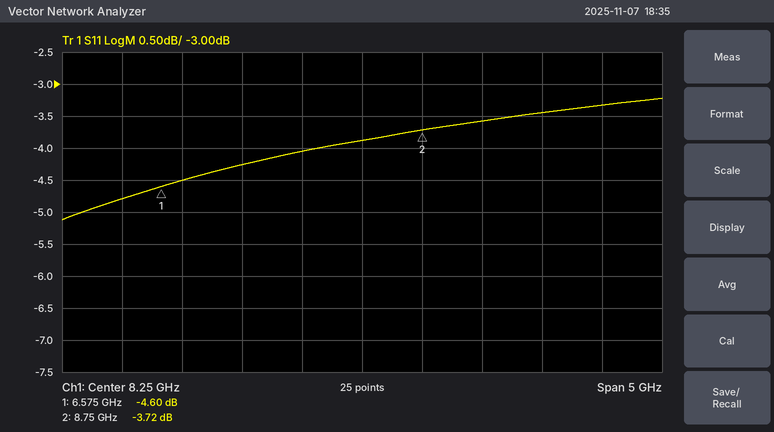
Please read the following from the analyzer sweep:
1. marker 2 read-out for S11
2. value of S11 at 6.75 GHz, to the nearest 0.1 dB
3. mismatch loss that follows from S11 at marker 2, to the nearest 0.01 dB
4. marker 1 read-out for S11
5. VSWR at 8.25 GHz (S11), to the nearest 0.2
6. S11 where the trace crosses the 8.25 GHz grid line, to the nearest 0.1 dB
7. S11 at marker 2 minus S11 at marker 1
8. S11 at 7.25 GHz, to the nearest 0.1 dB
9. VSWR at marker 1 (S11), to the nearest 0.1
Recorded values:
-3.72 dB
-4.5 dB
2.40 dB
-4.60 dB
4.6
-3.9 dB
0.88 dB
-4.3 dB
3.9
